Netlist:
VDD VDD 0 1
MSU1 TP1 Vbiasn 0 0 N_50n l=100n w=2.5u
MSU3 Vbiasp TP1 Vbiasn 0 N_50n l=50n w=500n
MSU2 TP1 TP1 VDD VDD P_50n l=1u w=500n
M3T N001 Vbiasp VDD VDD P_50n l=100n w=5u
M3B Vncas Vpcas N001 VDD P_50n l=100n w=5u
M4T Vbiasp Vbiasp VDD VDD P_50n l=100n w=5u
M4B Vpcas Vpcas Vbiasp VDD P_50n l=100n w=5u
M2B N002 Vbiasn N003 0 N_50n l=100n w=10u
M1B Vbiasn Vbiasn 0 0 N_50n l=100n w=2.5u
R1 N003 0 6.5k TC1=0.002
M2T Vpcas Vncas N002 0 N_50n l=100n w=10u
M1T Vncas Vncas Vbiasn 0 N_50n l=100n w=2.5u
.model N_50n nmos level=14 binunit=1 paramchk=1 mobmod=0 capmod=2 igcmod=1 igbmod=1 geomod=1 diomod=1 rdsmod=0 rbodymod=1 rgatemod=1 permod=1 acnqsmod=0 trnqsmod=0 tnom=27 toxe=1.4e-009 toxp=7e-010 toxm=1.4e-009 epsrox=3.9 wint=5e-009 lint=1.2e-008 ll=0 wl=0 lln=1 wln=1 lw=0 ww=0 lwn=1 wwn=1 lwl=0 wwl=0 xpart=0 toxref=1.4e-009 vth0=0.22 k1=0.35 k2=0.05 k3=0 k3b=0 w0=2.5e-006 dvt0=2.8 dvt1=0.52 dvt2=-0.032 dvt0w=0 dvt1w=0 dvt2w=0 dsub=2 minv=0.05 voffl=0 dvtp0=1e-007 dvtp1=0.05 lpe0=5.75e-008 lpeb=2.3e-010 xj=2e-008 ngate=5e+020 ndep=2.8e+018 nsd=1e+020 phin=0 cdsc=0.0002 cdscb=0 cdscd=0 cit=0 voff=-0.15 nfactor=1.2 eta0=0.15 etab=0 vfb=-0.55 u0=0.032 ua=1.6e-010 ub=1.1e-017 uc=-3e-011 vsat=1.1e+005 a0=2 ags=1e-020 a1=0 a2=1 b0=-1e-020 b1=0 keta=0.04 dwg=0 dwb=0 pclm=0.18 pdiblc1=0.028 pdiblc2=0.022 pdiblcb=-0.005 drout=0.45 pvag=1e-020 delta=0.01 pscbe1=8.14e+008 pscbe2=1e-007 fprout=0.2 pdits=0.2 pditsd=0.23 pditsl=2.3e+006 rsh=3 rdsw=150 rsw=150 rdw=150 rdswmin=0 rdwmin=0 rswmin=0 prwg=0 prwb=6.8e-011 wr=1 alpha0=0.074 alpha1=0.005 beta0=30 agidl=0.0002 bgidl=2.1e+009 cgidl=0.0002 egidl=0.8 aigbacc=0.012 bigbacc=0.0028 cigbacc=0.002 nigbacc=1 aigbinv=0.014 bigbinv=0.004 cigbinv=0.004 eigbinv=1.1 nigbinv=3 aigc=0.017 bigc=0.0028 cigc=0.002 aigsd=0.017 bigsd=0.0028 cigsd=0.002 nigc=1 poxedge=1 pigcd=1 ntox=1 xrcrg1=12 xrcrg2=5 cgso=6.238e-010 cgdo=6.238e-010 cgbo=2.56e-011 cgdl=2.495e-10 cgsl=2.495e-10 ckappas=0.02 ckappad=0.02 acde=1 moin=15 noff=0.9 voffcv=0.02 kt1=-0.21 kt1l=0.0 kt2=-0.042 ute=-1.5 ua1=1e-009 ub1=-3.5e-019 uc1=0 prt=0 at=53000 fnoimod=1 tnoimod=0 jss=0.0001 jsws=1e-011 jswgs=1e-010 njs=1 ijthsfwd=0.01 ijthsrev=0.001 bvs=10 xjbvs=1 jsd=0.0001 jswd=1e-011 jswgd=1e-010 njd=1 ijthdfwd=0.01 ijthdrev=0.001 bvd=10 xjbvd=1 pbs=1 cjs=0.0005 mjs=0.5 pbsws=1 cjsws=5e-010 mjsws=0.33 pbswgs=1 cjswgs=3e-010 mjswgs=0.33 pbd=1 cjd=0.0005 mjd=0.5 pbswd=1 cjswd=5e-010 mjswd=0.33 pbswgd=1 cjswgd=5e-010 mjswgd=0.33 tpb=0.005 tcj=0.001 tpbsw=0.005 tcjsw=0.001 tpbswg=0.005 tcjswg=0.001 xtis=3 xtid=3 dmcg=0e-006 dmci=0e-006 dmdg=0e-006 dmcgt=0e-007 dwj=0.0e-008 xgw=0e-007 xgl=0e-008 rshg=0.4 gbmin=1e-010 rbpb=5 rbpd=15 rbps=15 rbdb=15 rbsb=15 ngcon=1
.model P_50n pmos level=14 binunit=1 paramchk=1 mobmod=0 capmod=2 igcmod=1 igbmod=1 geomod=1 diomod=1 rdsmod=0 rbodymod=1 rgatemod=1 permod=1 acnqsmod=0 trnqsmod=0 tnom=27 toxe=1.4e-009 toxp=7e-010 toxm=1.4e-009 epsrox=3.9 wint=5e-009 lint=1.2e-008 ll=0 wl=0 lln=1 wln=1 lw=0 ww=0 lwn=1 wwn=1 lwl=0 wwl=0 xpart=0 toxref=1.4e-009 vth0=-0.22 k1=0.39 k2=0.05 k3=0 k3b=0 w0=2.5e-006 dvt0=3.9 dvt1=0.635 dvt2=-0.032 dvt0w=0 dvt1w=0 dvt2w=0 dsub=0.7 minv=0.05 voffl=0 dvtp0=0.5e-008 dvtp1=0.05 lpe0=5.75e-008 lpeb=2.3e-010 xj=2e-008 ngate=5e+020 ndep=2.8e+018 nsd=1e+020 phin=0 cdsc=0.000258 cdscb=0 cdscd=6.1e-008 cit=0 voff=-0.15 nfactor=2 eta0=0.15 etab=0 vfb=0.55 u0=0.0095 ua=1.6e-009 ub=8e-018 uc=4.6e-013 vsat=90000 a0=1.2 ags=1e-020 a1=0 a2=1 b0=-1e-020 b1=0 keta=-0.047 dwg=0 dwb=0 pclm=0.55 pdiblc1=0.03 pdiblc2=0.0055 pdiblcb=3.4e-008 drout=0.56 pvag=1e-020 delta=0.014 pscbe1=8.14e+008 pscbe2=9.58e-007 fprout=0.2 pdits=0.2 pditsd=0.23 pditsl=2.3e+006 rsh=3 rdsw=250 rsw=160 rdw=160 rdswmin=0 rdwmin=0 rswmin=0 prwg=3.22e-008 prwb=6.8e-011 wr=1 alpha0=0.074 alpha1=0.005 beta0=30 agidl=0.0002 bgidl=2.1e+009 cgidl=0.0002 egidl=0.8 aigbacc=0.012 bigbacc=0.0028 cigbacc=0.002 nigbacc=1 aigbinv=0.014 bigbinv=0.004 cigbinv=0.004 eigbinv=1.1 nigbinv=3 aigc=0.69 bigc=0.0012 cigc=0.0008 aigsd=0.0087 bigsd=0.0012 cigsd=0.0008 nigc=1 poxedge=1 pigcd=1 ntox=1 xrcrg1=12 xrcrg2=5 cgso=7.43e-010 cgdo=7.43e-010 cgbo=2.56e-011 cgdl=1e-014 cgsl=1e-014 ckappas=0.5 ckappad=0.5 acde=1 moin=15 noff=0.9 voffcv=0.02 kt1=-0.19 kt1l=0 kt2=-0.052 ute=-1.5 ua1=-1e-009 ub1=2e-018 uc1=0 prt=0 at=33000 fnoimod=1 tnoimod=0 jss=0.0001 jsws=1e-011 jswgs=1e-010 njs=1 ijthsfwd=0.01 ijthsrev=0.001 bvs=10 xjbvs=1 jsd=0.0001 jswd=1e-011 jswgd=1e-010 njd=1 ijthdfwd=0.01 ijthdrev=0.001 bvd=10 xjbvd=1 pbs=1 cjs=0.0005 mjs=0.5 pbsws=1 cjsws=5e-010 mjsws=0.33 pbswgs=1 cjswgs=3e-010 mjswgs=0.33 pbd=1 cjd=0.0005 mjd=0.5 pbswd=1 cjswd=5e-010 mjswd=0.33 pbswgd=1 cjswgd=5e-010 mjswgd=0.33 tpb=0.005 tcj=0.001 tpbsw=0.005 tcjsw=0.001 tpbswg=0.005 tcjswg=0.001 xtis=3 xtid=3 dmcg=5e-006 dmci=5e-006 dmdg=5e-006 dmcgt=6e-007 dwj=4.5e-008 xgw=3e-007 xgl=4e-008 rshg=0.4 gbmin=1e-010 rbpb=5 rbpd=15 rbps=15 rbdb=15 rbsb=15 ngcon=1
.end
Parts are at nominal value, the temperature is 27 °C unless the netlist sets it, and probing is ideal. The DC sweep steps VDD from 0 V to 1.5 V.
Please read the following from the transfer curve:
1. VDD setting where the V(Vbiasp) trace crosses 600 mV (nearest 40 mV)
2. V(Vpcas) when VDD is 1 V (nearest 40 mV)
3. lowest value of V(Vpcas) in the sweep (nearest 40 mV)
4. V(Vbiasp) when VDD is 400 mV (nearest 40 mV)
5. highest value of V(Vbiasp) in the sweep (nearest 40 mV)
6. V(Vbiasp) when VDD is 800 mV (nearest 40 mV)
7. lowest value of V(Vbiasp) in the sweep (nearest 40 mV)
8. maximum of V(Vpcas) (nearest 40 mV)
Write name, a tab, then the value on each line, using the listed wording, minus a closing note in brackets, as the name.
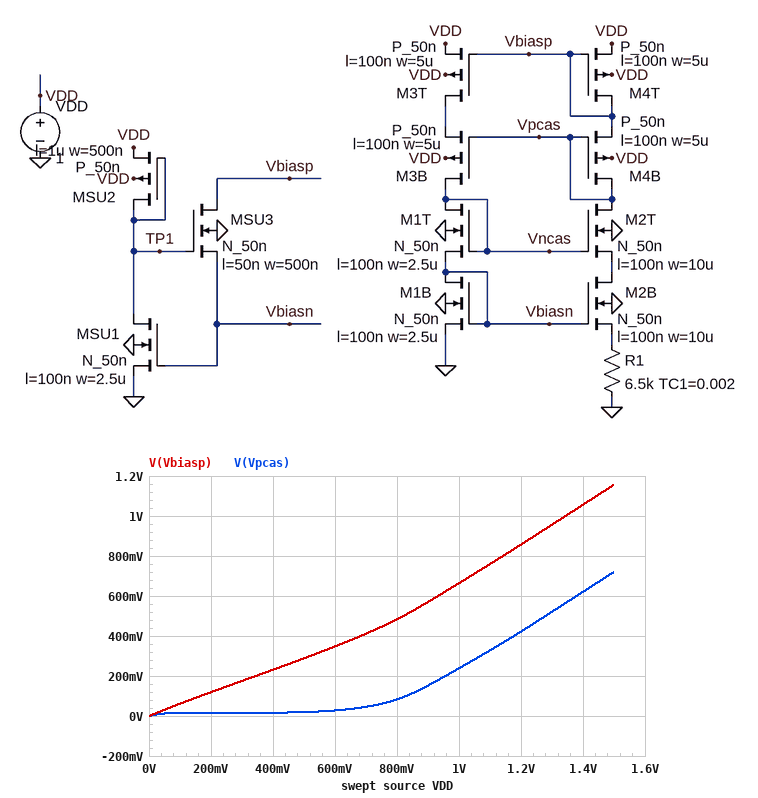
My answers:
VDD setting where the V(Vbiasp) trace crosses 600 mV	920 mV
V(Vpcas) when VDD is 1 V	240 mV
lowest value of V(Vpcas) in the sweep	0 V
V(Vbiasp) when VDD is 400 mV	240 mV
highest value of V(Vbiasp) in the sweep	1.16 V
V(Vbiasp) when VDD is 800 mV	480 mV
lowest value of V(Vbiasp) in the sweep	0 V
maximum of V(Vpcas)	720 mV
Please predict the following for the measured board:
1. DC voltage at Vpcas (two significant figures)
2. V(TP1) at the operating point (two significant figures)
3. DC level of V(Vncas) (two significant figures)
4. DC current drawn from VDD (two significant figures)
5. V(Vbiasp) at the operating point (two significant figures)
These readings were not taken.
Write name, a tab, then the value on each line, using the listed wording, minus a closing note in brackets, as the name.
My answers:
DC voltage at Vpcas	240 mV
V(TP1) at the operating point	59 mV
DC level of V(Vncas)	750 mV
DC current drawn from VDD	20 µA
V(Vbiasp) at the operating point	660 mV
